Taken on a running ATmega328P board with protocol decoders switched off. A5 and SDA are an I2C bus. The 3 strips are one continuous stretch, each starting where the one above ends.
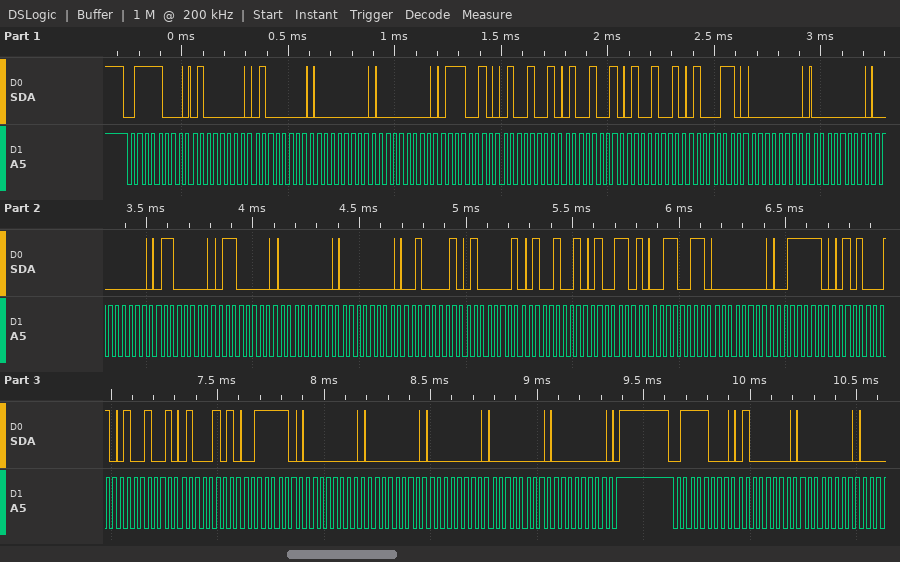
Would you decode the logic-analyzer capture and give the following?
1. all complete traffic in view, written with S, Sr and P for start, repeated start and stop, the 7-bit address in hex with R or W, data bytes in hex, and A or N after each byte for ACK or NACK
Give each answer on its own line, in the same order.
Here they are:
S 3CW A 40 A 40 A 00 A 00 A 72 A 49 A 49 A 49 A 46 A 00 A 00 A 00 A 60 A 60 A 00 A 00 A 21 A 41 A 49 A 4D A 33 A 00 A 3E A 51 A 49 A 45 A 3E A 00 A 00 A 00 A 00 A 00 A P S 3CW A 40 A 00 A
